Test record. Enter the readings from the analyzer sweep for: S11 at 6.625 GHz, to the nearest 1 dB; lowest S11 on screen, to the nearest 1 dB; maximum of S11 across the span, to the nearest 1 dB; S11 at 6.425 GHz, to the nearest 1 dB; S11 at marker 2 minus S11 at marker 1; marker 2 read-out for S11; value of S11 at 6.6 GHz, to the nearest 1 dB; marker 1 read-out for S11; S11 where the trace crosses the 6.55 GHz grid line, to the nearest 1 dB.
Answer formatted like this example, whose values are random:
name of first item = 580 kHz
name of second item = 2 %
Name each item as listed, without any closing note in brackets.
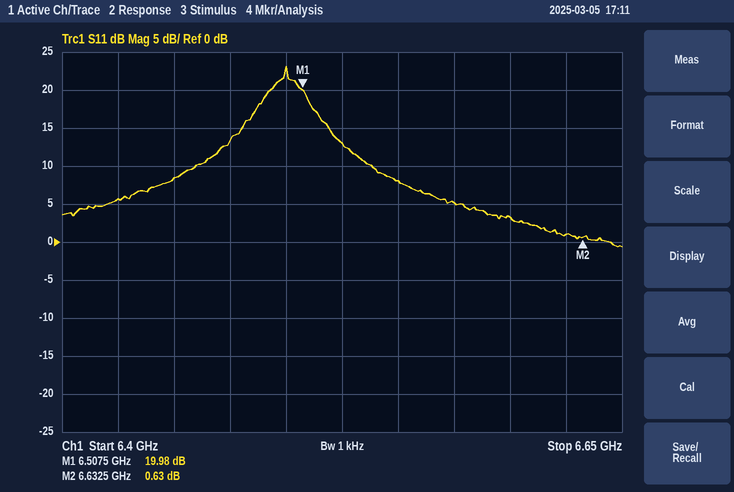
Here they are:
S11 at 6.625 GHz, to the nearest 1 dB = 1 dB
lowest S11 on screen, to the nearest 1 dB = -1 dB
maximum of S11 across the span, to the nearest 1 dB = 23 dB
S11 at 6.425 GHz, to the nearest 1 dB = 6 dB
S11 at marker 2 minus S11 at marker 1 = -19.35 dB
marker 2 read-out for S11 = 0.63 dB
value of S11 at 6.6 GHz, to the nearest 1 dB = 3 dB
marker 1 read-out for S11 = 19.98 dB
S11 where the trace crosses the 6.55 GHz grid line, to the nearest 1 dB = 8 dB
